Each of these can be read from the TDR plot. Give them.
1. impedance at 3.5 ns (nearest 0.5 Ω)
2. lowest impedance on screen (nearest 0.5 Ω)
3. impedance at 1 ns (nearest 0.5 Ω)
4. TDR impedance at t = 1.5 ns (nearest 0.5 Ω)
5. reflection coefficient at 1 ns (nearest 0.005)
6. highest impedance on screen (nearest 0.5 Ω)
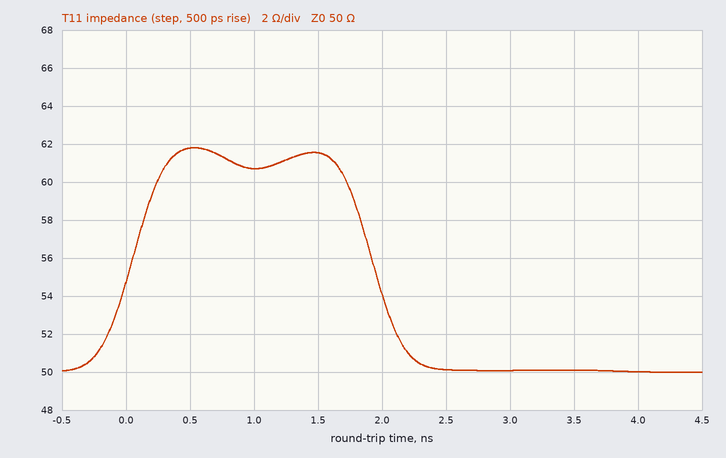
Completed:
50.0 Ω
50.0 Ω
60.5 Ω
61.5 Ω
+0.095
62.0 Ω
